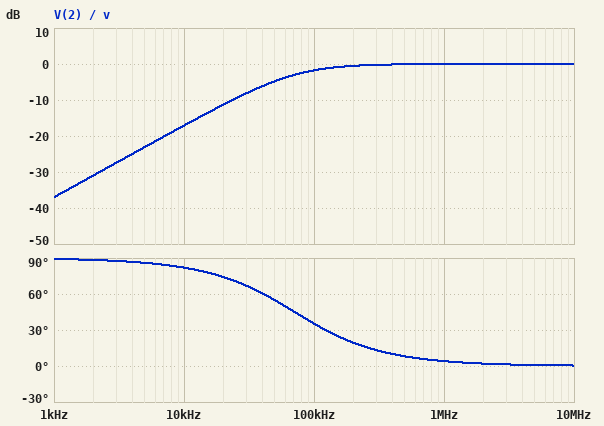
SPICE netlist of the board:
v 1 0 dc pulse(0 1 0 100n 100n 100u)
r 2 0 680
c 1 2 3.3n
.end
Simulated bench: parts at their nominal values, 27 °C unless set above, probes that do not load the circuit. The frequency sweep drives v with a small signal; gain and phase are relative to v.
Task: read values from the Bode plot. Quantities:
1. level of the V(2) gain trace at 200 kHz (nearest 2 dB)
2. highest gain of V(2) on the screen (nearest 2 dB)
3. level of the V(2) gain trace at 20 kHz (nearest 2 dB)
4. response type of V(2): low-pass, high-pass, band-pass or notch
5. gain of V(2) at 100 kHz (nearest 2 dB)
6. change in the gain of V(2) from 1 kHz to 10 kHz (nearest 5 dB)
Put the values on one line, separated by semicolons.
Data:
0 dB; 0 dB; -12 dB; high-pass; -2 dB; 20 dB
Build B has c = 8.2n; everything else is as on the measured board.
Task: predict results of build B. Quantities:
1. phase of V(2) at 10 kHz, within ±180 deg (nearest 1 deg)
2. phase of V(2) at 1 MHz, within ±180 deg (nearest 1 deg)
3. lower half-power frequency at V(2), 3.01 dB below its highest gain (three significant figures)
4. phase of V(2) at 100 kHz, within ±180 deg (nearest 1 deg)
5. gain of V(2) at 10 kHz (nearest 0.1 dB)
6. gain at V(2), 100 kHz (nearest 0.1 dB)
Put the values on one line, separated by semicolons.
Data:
71 deg; 2 deg; 28.5 kHz; 16 deg; -9.6 dB; -0.3 dB
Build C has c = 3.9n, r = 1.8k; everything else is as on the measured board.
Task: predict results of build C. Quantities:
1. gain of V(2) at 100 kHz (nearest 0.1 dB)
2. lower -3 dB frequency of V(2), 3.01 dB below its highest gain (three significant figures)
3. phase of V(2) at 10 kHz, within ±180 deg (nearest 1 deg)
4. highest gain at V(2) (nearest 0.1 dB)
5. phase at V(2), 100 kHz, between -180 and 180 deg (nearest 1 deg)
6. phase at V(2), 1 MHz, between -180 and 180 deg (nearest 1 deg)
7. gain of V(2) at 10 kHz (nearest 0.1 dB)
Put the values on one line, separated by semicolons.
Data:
-0.2 dB; 22.7 kHz; 66 deg; 0 dB; 13 deg; 1 deg; -7.9 dB
